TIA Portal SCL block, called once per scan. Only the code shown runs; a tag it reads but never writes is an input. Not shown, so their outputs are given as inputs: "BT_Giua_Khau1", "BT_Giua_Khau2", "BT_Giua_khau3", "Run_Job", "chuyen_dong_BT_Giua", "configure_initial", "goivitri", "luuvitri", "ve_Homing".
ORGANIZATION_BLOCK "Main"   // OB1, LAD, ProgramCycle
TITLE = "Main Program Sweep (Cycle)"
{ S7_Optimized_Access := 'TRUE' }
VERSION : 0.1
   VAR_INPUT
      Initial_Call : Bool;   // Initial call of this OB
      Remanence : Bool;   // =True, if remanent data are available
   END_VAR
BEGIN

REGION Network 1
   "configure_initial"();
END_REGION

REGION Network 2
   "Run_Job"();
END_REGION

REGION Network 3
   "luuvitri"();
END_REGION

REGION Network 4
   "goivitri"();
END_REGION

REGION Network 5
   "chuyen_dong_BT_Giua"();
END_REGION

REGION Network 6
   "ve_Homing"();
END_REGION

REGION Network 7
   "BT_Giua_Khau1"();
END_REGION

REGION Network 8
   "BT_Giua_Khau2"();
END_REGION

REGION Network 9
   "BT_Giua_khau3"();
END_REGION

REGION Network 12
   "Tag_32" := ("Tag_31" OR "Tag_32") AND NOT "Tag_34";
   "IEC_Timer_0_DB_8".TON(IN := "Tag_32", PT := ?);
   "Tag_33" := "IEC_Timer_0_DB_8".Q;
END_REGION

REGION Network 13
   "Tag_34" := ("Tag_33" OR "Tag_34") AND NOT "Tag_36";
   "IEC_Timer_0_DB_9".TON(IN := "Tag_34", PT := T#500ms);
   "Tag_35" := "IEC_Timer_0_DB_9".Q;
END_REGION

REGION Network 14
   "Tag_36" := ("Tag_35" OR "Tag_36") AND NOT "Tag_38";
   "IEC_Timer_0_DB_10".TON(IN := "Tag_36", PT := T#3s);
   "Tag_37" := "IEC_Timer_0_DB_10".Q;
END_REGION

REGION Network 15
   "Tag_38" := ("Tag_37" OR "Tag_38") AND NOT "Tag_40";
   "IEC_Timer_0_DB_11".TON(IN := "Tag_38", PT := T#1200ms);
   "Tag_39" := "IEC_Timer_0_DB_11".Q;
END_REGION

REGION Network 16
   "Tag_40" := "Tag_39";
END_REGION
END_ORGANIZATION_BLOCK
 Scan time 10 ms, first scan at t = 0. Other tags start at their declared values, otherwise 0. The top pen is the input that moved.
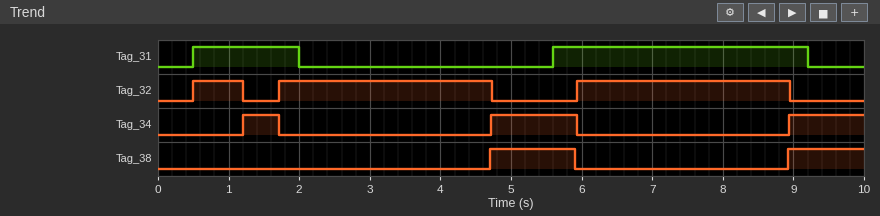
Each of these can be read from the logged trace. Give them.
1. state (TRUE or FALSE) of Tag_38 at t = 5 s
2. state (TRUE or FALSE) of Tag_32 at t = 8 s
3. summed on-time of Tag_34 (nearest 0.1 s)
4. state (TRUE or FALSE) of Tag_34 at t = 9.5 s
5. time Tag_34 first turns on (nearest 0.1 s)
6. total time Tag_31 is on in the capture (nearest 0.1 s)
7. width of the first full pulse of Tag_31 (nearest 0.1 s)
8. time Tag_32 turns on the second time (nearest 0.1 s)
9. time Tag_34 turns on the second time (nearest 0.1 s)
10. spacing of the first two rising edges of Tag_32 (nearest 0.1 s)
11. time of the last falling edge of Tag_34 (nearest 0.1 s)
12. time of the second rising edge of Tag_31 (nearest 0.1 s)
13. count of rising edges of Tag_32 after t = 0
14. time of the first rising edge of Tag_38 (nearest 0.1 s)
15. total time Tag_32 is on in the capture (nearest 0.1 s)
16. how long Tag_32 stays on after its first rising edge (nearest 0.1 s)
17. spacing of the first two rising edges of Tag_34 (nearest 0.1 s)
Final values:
TRUE
TRUE
2.8 s
TRUE
1.2 s
5.1 s
1.5 s
1.7 s
4.7 s
1.2 s
5.9 s
5.6 s
3
4.7 s
6.7 s
0.7 s
3.5 s
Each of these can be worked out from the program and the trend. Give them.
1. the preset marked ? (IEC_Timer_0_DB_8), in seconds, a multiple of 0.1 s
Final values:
0.7 s
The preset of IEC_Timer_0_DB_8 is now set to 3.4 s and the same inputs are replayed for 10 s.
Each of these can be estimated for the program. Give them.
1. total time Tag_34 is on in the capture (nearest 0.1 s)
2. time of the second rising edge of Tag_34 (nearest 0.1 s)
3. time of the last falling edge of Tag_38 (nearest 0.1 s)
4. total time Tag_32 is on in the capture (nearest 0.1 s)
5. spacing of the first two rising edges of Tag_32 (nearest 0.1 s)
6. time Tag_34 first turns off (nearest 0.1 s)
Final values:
1.0 s
9.0 s
8.6 s
6.8 s
5.1 s
4.4 s
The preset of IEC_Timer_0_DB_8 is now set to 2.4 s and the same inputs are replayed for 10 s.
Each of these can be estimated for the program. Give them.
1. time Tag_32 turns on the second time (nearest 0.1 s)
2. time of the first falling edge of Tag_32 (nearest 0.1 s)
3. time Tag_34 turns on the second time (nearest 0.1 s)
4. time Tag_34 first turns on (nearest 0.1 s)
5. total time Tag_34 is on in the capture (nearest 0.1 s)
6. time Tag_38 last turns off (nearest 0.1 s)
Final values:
5.6 s
2.9 s
8.0 s
2.9 s
1.0 s
7.6 s
